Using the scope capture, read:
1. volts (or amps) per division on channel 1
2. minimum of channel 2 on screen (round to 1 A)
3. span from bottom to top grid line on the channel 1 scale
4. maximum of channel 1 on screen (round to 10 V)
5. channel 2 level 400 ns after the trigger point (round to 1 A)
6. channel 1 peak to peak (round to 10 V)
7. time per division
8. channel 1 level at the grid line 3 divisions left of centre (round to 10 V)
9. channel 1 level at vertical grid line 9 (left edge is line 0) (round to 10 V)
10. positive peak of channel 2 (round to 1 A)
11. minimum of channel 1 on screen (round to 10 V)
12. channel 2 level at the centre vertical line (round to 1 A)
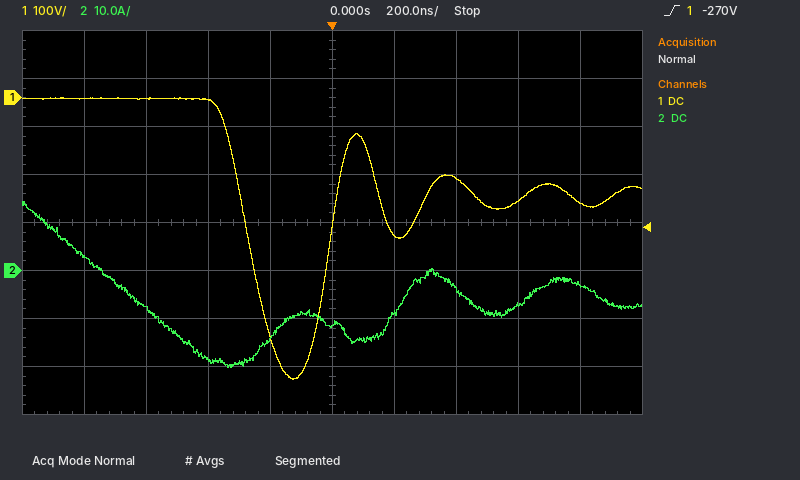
100 V
-20 A
800 V
0 V
-4 A
590 V
200 ns
0 V
-220 V
14 A
-590 V
-11 A
